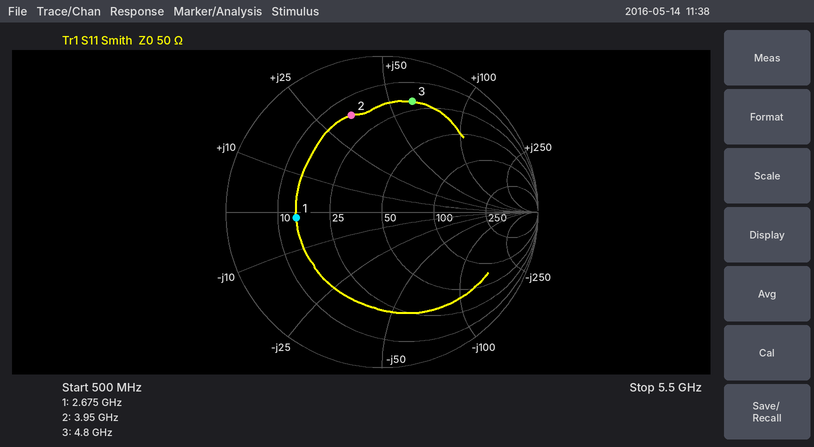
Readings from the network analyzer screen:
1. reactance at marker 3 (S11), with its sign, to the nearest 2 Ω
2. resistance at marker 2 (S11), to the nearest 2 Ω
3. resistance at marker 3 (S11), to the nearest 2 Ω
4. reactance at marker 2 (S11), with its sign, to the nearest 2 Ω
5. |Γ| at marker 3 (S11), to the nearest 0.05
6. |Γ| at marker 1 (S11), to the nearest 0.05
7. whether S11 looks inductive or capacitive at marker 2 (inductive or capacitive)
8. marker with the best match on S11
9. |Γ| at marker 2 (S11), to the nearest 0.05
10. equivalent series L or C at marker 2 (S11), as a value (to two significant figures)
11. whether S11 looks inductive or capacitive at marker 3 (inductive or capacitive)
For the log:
+62 Ω
16 Ω
20 Ω
+34 Ω
0.75
0.55
inductive
marker 1
0.65
1.4 nH
inductive
